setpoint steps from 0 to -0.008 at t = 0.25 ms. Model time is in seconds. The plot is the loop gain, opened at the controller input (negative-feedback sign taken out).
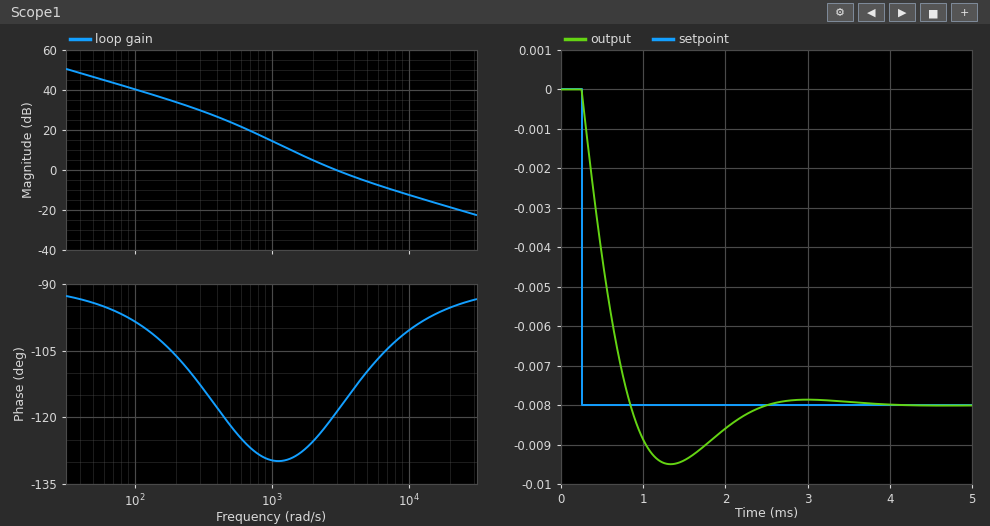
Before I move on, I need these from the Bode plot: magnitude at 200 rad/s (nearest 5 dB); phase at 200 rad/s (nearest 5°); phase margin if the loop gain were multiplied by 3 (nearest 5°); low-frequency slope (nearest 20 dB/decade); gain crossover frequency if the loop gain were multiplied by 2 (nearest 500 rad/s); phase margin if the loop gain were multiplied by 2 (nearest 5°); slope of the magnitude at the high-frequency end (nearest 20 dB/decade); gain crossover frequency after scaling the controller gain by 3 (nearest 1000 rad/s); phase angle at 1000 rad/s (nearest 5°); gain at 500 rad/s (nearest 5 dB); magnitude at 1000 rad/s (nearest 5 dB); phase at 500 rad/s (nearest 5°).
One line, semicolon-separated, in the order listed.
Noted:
35 dB; -105°; 75°; -20 dB/decade; 5000 rad/s; 70°; -20 dB/decade; 7000 rad/s; -130°; 25 dB; 15 dB; -120°
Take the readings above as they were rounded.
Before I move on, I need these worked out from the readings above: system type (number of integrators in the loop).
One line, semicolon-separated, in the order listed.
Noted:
1
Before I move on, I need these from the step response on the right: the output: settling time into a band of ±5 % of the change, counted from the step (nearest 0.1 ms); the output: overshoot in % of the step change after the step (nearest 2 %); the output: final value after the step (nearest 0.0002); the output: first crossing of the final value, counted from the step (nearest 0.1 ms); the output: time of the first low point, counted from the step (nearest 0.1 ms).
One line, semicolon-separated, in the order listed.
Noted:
1.9 ms; 18 %; -0.0080; 0.6 ms; 1.1 ms
